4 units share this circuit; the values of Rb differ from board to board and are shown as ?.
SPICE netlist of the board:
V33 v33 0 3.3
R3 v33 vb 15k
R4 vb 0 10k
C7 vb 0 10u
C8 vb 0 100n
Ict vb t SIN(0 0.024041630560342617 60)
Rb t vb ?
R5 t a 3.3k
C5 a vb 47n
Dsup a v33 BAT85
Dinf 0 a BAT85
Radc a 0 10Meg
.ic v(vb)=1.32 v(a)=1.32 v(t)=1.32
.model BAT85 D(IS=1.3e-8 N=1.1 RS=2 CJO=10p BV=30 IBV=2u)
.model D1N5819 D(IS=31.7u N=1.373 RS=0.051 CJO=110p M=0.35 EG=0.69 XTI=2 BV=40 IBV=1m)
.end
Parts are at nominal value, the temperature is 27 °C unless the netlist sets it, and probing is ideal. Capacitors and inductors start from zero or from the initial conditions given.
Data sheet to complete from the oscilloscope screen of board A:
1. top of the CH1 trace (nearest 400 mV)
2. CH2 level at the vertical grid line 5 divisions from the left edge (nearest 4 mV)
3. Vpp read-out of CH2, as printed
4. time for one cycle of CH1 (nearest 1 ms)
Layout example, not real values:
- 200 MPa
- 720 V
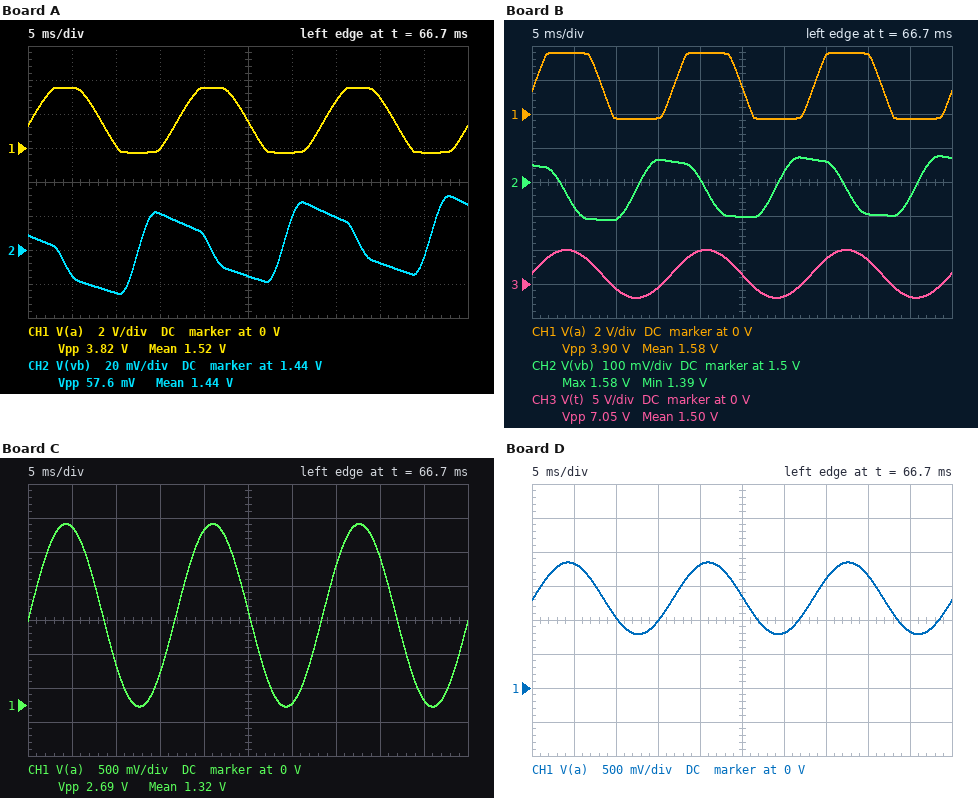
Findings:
- 3.6 V
- 1.424 V
- 57.6 mV
- 17 ms
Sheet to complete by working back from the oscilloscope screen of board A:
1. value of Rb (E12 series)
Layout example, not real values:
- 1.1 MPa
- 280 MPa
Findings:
- 100 Ω
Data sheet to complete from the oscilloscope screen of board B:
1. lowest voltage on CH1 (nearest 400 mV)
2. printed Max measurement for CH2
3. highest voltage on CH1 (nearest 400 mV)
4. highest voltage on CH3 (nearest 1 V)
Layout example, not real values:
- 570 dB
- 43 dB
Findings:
- -400 mV
- 1.58 V
- 3.6 V
- 5 V
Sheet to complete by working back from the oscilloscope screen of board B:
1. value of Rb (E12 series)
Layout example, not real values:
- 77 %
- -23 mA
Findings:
- 150 Ω
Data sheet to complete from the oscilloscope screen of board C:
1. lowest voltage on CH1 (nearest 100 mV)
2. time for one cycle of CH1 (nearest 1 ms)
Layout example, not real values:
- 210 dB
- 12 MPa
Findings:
- 0 V
- 17 ms
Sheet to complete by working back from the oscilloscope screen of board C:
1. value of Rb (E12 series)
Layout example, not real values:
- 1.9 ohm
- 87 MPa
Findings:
- 56 Ω
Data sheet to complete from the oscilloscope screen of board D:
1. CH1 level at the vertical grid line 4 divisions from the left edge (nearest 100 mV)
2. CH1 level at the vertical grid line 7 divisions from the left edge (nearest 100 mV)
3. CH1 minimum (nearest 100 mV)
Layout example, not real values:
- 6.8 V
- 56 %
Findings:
- 1.8 V
- 1.6 V
- 800 mV
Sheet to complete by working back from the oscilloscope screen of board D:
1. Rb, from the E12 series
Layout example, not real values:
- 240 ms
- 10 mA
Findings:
- 22 Ω
